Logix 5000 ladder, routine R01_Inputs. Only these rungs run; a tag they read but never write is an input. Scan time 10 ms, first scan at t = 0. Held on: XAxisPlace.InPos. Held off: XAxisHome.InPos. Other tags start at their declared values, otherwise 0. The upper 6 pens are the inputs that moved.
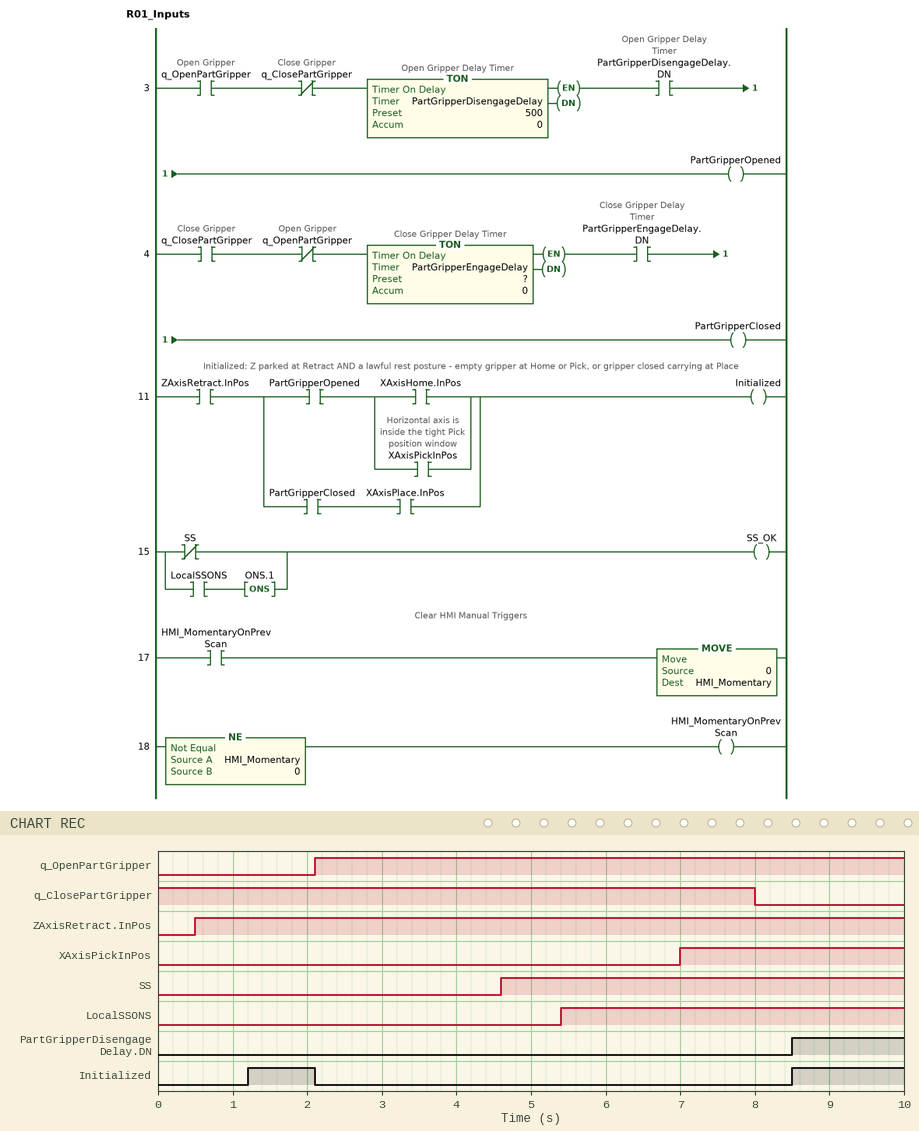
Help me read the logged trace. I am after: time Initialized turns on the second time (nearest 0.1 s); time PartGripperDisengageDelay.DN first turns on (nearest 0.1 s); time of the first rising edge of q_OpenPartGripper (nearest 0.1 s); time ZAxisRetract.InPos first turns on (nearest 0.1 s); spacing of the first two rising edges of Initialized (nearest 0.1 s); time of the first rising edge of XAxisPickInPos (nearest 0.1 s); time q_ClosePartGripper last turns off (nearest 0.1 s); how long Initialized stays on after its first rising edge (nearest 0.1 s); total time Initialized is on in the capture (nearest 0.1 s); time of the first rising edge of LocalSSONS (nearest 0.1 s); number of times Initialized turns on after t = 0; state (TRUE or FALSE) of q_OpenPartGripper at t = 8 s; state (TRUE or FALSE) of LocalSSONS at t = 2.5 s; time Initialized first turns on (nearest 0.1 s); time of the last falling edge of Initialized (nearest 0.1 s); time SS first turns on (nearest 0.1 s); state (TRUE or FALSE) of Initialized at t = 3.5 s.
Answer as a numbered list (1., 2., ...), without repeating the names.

1. 8.5 s
2. 8.5 s
3. 2.1 s
4. 0.5 s
5. 7.3 s
6. 7.0 s
7. 8.0 s
8. 0.9 s
9. 2.4 s
10. 5.4 s
11. 2
12. TRUE
13. FALSE
14. 1.2 s
15. 2.1 s
16. 4.6 s
17. FALSE
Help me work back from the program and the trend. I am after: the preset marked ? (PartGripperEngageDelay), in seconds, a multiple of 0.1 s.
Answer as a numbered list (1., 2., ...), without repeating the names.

1. 1.2 s
